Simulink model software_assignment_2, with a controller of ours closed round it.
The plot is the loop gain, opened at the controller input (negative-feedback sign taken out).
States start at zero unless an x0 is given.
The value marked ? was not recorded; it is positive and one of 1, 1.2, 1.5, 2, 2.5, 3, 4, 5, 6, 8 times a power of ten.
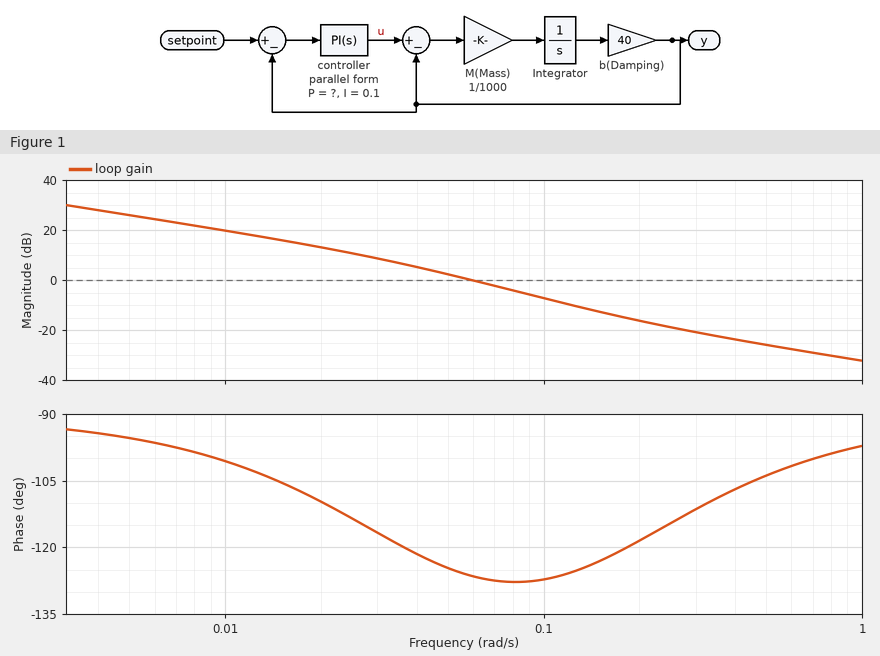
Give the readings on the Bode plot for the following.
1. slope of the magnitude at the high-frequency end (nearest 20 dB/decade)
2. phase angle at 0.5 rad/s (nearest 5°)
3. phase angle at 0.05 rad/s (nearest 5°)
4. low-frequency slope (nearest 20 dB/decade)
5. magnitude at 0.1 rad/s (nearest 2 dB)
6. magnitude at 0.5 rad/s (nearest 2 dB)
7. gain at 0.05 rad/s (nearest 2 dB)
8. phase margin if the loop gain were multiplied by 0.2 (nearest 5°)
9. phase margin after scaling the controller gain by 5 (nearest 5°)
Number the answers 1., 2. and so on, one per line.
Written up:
1. -20 dB/decade
2. -105°
3. -125°
4. -20 dB/decade
5. -8 dB
6. -26 dB
7. 2 dB
8. 70°
9. 60°
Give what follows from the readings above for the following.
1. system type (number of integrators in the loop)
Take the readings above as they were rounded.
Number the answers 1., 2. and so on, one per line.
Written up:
1. 1
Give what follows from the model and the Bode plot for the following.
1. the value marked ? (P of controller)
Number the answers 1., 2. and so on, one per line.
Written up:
1. 0.6
